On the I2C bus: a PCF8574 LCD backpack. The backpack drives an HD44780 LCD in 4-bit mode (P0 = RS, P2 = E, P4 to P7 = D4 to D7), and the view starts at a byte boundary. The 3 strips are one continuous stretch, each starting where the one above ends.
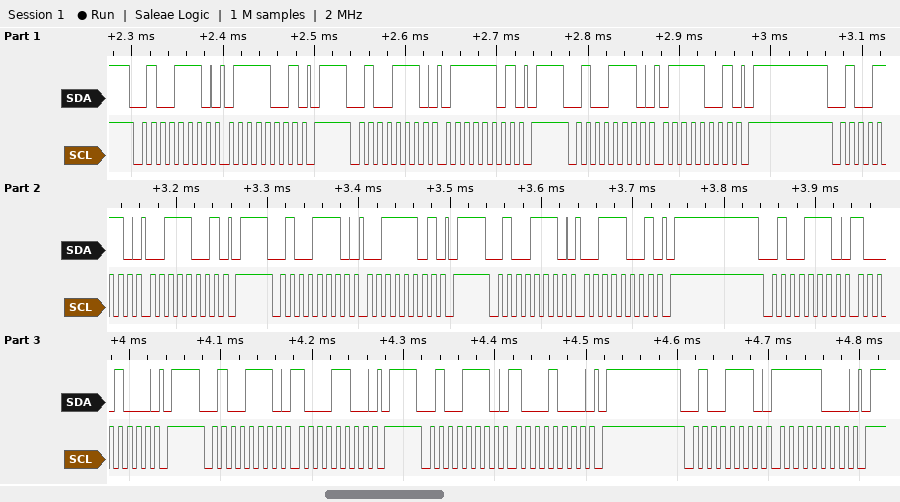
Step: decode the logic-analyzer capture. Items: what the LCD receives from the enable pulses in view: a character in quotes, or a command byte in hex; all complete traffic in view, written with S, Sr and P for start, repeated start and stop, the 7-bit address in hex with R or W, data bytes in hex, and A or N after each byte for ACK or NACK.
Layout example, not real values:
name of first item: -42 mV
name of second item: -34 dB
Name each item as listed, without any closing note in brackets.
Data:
what the LCD receives from the enable pulses in view: a character in quotes, or a command byte in hex: 's'
all complete traffic in view, written with S, Sr and P for start, repeated start and stop, the 7-bit address in hex with R or W, data bytes in hex, and A or N after each byte for ACK or NACK: S 27W A 79 A P S 27W A 7D A P S 27W A 79 A P S 27W A 39 A P S 27W A 3D A P S 27W A 39 A P S 27W A 88 A P S 27W A 8C A P S 27W A 88 A P S 27W A F8 A P
